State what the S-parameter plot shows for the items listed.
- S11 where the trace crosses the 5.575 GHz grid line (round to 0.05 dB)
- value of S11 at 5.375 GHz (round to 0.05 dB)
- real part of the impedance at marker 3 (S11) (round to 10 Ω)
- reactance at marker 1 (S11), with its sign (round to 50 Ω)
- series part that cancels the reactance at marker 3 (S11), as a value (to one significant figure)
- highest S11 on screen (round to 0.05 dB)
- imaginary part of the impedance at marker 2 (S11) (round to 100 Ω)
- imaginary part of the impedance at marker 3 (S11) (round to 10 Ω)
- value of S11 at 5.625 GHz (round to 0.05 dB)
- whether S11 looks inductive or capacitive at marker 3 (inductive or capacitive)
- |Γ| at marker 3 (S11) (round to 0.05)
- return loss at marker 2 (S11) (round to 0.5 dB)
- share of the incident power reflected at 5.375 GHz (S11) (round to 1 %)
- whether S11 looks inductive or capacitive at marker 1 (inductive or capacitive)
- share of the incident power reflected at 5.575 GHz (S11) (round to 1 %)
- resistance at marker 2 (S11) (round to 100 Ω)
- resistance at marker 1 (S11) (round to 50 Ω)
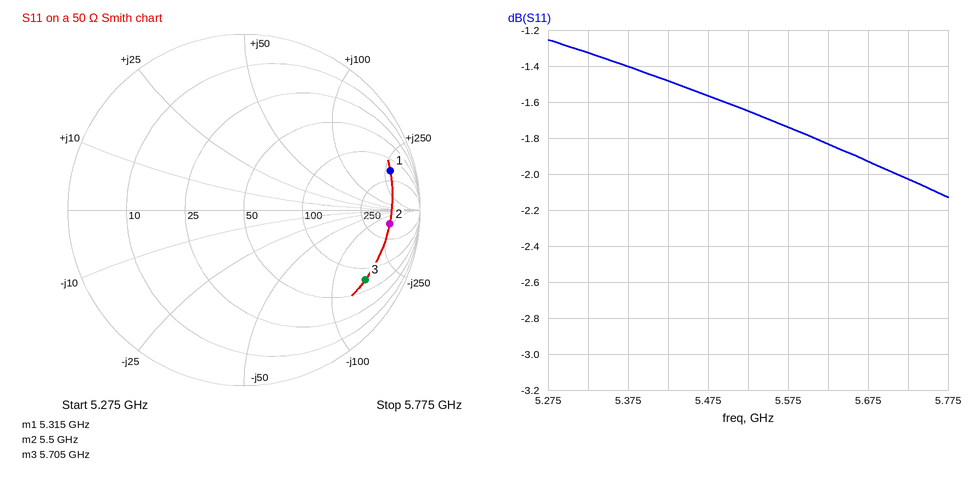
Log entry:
-1.75 dB
-1.40 dB
70 Ω
+300 Ω
4 nH
-1.25 dB
-200 Ω
-160 Ω
-1.85 dB
capacitive
0.80
1.5 dB
72 %
inductive
67 %
400 Ω
150 Ω
